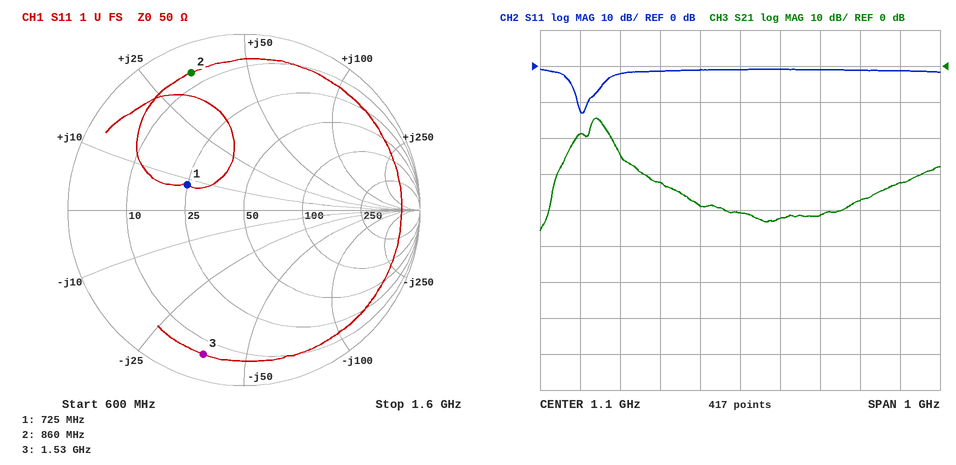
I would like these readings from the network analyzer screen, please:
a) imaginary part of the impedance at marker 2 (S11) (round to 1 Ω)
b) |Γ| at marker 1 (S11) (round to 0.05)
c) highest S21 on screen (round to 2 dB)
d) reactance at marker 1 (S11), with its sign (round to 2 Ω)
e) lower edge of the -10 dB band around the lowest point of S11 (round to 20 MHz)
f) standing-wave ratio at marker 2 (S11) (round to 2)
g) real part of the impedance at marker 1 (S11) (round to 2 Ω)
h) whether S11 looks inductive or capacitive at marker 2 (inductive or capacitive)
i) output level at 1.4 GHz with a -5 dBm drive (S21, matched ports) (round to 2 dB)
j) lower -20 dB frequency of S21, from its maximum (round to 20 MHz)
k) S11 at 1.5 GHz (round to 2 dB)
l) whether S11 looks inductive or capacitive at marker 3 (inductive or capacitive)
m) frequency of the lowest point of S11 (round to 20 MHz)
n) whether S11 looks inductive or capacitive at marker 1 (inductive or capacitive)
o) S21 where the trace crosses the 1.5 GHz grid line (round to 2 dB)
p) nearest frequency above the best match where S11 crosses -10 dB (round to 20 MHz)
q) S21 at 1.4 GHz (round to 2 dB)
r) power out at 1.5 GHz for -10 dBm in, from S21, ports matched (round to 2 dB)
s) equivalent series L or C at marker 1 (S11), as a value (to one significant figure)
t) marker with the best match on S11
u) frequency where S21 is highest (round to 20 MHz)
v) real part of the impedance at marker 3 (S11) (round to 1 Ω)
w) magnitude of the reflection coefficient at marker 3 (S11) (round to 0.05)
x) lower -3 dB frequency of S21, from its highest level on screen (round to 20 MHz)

+34 Ω
0.35
-14 dB
+8 Ω
700 MHz
12
24 Ω
inductive
-42 dBm
640 MHz
-2 dB
capacitive
700 MHz
inductive
-32 dB
720 MHz
-38 dB
-42 dBm
2 nH
marker 1
740 MHz
6 Ω
0.85
720 MHz
